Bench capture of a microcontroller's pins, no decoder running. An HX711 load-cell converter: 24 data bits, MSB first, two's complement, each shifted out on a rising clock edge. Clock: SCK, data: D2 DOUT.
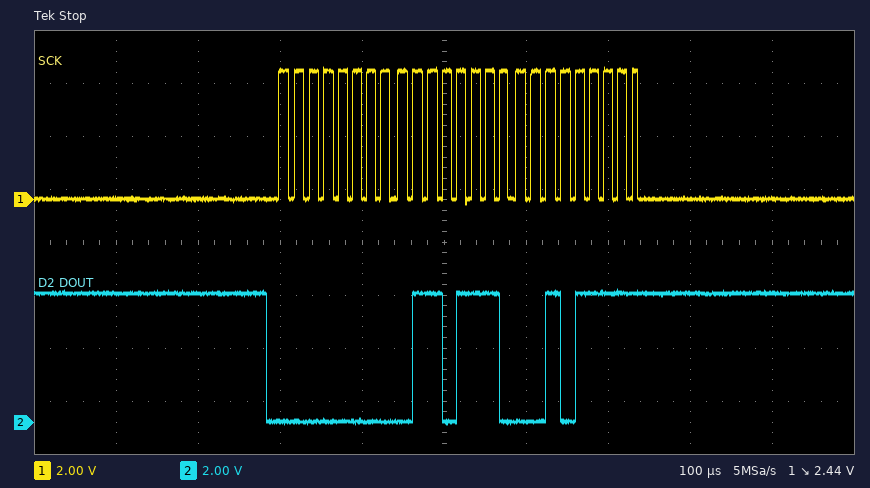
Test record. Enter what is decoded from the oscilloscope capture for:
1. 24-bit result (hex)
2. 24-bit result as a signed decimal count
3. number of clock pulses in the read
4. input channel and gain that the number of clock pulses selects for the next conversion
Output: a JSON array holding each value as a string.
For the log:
["0x006E2F", "28207", "25", "channel A, gain 128"]
